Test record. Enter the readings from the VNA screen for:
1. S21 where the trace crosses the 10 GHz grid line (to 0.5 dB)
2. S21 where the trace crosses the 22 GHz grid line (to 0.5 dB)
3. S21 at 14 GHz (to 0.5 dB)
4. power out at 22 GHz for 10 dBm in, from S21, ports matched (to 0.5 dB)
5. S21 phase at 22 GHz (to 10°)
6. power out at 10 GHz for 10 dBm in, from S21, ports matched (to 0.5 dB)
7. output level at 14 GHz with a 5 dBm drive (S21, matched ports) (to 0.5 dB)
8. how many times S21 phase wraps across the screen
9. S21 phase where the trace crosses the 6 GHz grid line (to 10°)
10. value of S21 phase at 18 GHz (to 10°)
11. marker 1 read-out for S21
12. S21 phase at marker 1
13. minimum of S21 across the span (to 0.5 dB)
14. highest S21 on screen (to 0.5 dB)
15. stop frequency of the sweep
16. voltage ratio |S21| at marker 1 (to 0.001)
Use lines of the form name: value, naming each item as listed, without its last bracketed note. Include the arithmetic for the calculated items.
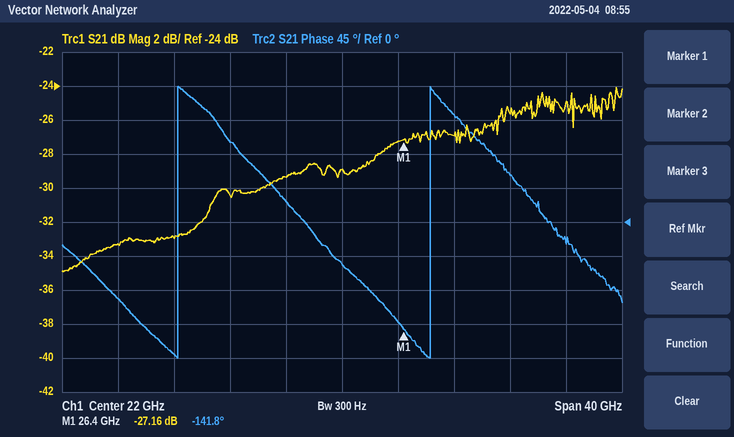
S21 where the trace crosses the 10 GHz grid line: -33.0 dB
S21 where the trace crosses the 22 GHz grid line: -29.0 dB
S21 at 14 GHz: -30.5 dB
power out at 22 GHz for 10 dBm in, from S21, ports matched: 10 dBm + (-29.0 dB) = -19.0 dBm
S21 phase at 22 GHz: -60°
power out at 10 GHz for 10 dBm in, from S21, ports matched: 10 dBm + (-33.0 dB) = -23.0 dBm
output level at 14 GHz with a 5 dBm drive (S21, matched ports): 5 dBm + (-30.5 dB) = -25.5 dBm
how many times S21 phase wraps across the screen: 2
S21 phase where the trace crosses the 6 GHz grid line: -100°
value of S21 phase at 18 GHz: 30°
marker 1 read-out for S21: -27.16 dB
S21 phase at marker 1: -141.8°
minimum of S21 across the span: -35.0 dB
highest S21 on screen: -24.0 dB
stop frequency of the sweep: 42 GHz
voltage ratio |S21| at marker 1: 10^(-27.16/20) ≈ 0.044
